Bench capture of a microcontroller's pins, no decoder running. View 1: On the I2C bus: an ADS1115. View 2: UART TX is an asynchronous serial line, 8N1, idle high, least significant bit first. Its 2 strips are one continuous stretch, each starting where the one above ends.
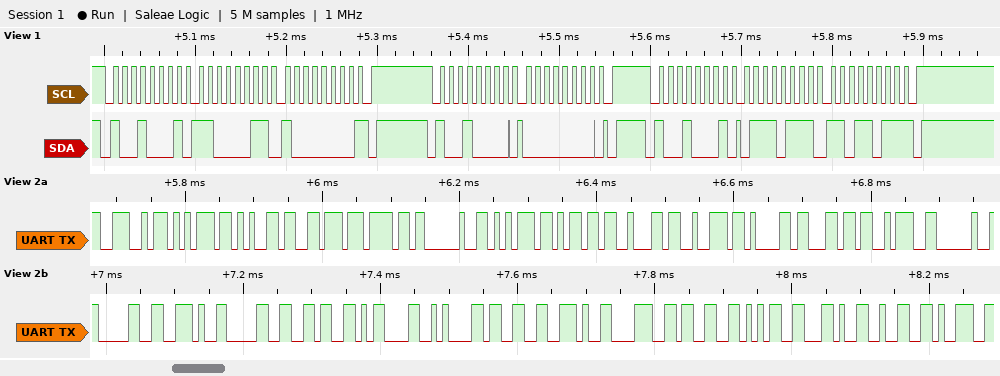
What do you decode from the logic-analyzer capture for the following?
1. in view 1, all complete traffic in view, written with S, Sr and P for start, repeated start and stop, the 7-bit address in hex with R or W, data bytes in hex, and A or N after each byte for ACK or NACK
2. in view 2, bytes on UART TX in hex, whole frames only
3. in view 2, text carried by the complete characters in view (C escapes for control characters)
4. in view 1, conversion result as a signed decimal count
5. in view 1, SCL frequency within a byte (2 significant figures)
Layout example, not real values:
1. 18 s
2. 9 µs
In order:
1. S 48R A C3 A 80 N P S 48W A 00 A P S 48R A 77 A DB N P
2. 4E 75 65 76 6F 20 75 6D 62 72 61 6C 3A 20 30 2E 30 36 0D 0A 33 2E 38 33 35 2C 32 39
3. "Nuevo umbral: 0.06\r\n3.835,29"
4. 30683
5. 100 kHz
